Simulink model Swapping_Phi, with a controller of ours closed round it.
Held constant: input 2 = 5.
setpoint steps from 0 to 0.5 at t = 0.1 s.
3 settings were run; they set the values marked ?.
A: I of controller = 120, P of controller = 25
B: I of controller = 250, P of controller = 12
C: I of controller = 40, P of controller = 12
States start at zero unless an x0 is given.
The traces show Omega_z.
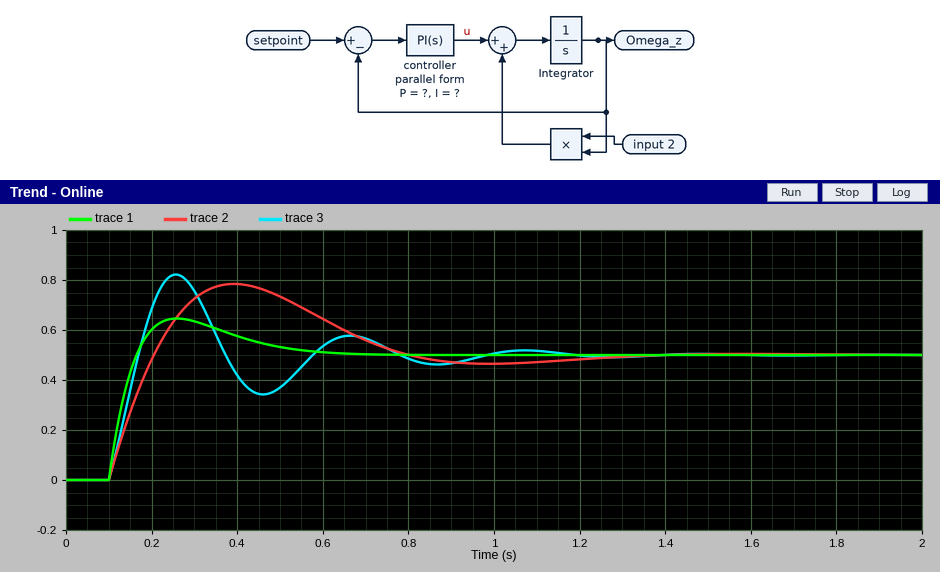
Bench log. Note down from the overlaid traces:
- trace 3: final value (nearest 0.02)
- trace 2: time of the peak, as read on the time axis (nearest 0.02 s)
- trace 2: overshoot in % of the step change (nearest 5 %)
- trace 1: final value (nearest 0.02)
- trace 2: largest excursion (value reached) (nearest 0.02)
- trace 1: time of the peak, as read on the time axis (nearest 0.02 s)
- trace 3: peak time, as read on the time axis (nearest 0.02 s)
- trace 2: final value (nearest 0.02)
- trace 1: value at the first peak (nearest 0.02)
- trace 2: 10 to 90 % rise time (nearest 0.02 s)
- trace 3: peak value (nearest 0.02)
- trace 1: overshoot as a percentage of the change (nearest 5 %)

0.50
0.40 s
55 %
0.50
0.78
0.26 s
0.26 s
0.50
0.64
0.08 s
0.82
30 %
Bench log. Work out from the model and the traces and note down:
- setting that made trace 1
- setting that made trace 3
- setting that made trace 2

A
B
C
